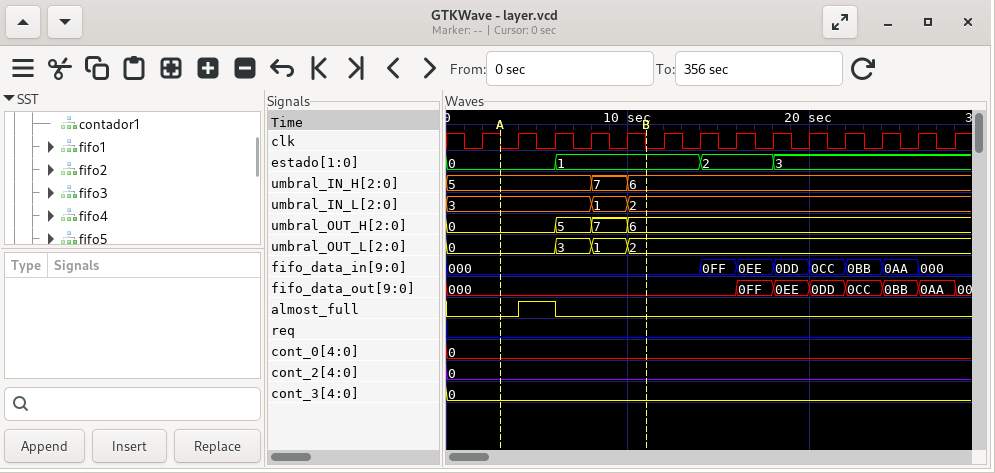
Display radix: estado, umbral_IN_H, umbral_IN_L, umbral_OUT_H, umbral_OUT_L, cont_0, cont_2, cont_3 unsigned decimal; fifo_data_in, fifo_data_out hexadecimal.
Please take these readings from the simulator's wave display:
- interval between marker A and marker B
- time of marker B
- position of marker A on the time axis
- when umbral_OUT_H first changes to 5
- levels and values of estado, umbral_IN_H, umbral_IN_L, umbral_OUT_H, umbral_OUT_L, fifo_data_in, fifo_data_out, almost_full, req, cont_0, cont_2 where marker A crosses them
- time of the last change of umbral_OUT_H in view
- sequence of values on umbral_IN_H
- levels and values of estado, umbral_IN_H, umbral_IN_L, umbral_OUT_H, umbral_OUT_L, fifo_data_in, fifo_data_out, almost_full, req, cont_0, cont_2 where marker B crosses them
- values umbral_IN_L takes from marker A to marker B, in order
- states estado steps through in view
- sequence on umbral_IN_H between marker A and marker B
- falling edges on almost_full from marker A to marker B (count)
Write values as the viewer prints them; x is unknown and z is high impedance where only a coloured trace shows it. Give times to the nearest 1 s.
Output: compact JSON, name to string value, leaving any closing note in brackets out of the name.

{"interval between marker A and marker B": "8 s", "time of marker B": "11 s", "position of marker A on the time axis": "3 s", "when umbral_OUT_H first changes to 5": "6 s", "levels and values of estado, umbral_IN_H, umbral_IN_L, umbral_OUT_H, umbral_OUT_L, fifo_data_in, fifo_data_out, almost_full, req, cont_0, cont_2 where marker A crosses them": "estado=0, umbral_IN_H=5, umbral_IN_L=3, umbral_OUT_H=0, umbral_OUT_L=0, fifo_data_in=000, fifo_data_out=000, almost_full=0, req=0, cont_0=0, cont_2=0", "time of the last change of umbral_OUT_H in view": "10 s", "sequence of values on umbral_IN_H": "5, 7, 6", "levels and values of estado, umbral_IN_H, umbral_IN_L, umbral_OUT_H, umbral_OUT_L, fifo_data_in, fifo_data_out, almost_full, req, cont_0, cont_2 where marker B crosses them": "estado=1, umbral_IN_H=6, umbral_IN_L=2, umbral_OUT_H=6, umbral_OUT_L=2, fifo_data_in=000, fifo_data_out=000, almost_full=0, req=0, cont_0=0, cont_2=0", "values umbral_IN_L takes from marker A to marker B, in order": "3, 1, 2", "states estado steps through in view": "0, 1, 2, 3", "sequence on umbral_IN_H between marker A and marker B": "5, 7, 6", "falling edges on almost_full from marker A to marker B": "1"}
